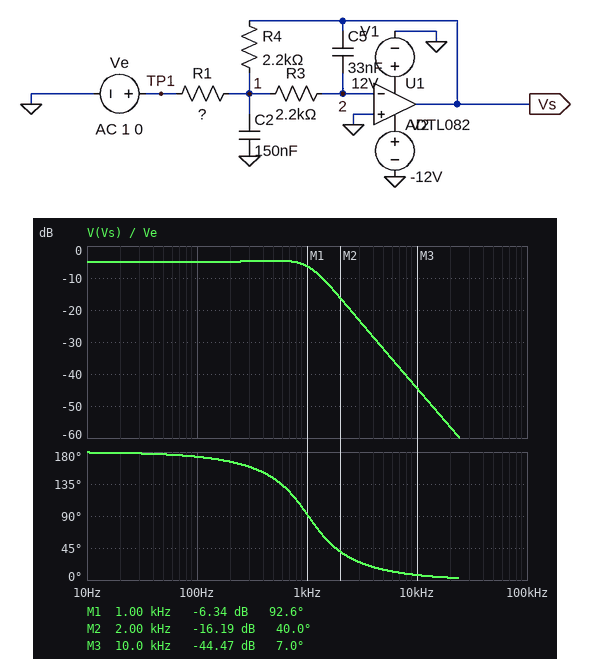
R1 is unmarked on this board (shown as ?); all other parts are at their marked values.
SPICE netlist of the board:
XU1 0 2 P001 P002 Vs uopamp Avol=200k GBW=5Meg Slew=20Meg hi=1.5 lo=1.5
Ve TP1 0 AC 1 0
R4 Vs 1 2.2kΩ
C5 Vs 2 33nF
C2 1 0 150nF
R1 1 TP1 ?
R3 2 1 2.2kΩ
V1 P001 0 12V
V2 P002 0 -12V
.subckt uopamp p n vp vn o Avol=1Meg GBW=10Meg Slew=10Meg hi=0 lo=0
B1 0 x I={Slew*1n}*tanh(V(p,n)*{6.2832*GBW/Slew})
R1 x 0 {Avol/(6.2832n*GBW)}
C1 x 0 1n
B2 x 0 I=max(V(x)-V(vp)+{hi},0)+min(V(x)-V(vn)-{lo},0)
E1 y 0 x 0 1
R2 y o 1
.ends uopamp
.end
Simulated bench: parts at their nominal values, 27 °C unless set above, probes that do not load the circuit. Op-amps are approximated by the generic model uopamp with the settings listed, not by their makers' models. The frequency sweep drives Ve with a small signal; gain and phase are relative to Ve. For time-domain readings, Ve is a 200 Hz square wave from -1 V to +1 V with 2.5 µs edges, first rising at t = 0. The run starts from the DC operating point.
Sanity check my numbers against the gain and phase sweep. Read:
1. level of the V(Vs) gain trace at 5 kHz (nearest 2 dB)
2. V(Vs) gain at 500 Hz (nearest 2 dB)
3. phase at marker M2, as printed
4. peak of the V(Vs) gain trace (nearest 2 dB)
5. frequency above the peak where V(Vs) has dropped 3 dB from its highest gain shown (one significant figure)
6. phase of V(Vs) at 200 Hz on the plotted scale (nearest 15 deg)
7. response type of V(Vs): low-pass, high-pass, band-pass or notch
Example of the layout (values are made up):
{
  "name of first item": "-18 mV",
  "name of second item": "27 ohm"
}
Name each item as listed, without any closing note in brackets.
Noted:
{
  "level of the V(Vs) gain trace at 5 kHz": "-32 dB",
  "V(Vs) gain at 500 Hz": "-4 dB",
  "phase at marker M2, as printed": "40.0 deg",
  "peak of the V(Vs) gain trace": "-4 dB",
  "frequency above the peak where V(Vs) has dropped 3 dB from its highest gain shown": "1 kHz",
  "phase of V(Vs) at 200 Hz on the plotted scale": "165 deg",
  "response type of V(Vs): low-pass, high-pass, band-pass or notch": "low-pass"
}
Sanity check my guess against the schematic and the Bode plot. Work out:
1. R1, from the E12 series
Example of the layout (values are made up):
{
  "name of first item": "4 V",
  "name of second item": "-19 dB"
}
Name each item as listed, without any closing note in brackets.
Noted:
{
  "R1, from the E12 series": "3.9 kΩ"
}
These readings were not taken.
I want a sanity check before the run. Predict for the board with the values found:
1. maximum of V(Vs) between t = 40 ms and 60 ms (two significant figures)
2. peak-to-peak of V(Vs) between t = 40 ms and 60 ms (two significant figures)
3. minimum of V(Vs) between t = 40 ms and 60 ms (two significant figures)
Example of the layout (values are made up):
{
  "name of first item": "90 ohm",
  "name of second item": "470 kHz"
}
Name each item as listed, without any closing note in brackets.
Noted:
{
  "maximum of V(Vs) between t = 40 ms and 60 ms": "670 mV",
  "peak-to-peak of V(Vs) between t = 40 ms and 60 ms": "1.3 V",
  "minimum of V(Vs) between t = 40 ms and 60 ms": "-670 mV"
}
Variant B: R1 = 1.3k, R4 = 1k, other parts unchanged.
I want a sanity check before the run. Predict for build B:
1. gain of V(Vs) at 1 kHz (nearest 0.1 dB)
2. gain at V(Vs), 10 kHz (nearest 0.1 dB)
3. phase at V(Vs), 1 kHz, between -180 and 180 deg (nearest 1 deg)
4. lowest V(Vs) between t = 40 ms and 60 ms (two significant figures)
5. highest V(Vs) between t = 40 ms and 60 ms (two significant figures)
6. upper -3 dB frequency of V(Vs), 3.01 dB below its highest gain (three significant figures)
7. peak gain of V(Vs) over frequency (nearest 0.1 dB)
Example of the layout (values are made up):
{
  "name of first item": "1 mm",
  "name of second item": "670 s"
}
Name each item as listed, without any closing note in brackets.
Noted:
{
  "gain of V(Vs) at 1 kHz": "-3.6 dB",
  "gain at V(Vs), 10 kHz": "-35.0 dB",
  "phase at V(Vs), 1 kHz, between -180 and 180 deg": "119 deg",
  "lowest V(Vs) between t = 40 ms and 60 ms": "-800 mV",
  "highest V(Vs) between t = 40 ms and 60 ms": "800 mV",
  "upper -3 dB frequency of V(Vs), 3.01 dB below its highest gain": "1.38 kHz",
  "peak gain of V(Vs) over frequency": "-2.3 dB"
}
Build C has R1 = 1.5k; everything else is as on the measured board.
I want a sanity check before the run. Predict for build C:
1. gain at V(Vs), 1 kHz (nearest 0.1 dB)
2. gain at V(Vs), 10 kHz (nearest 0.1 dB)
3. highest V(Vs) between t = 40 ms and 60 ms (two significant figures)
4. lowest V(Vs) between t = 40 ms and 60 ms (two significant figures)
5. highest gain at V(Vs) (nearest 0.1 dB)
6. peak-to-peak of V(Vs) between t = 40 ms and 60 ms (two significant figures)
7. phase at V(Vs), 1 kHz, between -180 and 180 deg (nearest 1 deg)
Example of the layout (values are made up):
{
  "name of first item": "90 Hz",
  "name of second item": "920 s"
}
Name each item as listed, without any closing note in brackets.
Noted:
{
  "gain at V(Vs), 1 kHz": "-0.7 dB",
  "gain at V(Vs), 10 kHz": "-36.2 dB",
  "highest V(Vs) between t = 40 ms and 60 ms": "1.5 V",
  "lowest V(Vs) between t = 40 ms and 60 ms": "-1.5 V",
  "highest gain at V(Vs)": "3.3 dB",
  "peak-to-peak of V(Vs) between t = 40 ms and 60 ms": "3.0 V",
  "phase at V(Vs), 1 kHz, between -180 and 180 deg": "92 deg"
}
